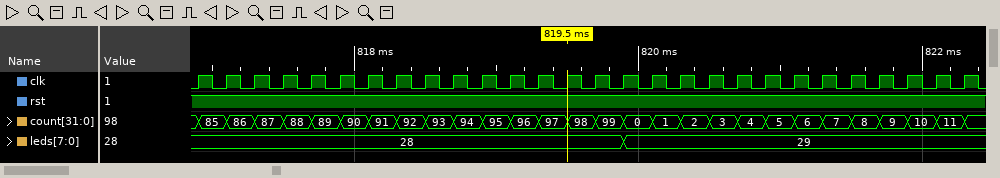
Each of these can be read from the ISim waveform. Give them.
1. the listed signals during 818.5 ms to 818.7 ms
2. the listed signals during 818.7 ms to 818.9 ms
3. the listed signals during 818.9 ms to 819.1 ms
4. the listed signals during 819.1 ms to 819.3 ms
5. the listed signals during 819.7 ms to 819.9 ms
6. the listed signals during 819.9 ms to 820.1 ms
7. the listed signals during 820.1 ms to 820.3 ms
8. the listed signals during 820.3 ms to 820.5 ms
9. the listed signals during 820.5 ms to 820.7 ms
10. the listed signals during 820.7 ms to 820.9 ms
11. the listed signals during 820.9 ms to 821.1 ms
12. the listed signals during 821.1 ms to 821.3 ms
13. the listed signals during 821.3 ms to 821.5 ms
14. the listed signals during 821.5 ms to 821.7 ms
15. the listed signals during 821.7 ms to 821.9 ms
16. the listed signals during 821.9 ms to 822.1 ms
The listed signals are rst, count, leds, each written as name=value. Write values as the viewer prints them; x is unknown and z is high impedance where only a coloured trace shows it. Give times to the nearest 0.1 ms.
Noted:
rst=1, count=93, leds=28
rst=1, count=94, leds=28
rst=1, count=95, leds=28
rst=1, count=96, leds=28
rst=1, count=99, leds=28
rst=1, count=0, leds=29
rst=1, count=1, leds=29
rst=1, count=2, leds=29
rst=1, count=3, leds=29
rst=1, count=4, leds=29
rst=1, count=5, leds=29
rst=1, count=6, leds=29
rst=1, count=7, leds=29
rst=1, count=8, leds=29
rst=1, count=9, leds=29
rst=1, count=10, leds=29
